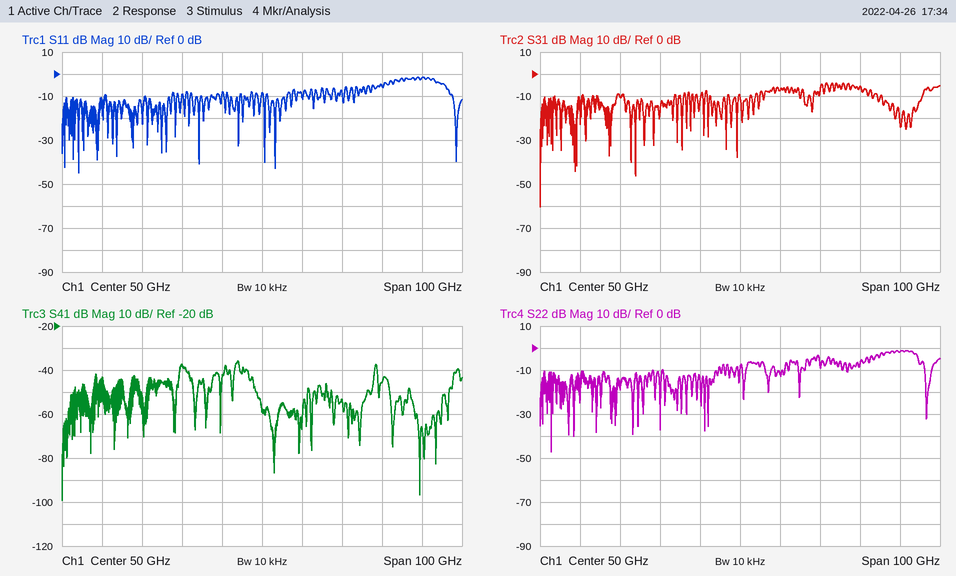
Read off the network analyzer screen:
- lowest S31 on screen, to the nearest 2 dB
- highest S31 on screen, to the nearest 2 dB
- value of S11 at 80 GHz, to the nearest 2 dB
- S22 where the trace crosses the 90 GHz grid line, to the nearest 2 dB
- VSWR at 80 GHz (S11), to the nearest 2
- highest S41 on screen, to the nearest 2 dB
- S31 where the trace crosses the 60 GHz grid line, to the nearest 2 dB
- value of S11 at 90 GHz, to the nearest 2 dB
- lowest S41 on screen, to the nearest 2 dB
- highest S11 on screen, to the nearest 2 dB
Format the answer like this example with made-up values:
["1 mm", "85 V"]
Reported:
["-60 dB", "-4 dB", "-6 dB", "-2 dB", "4", "-36 dB", "-8 dB", "-2 dB", "-100 dB", "-2 dB"]
